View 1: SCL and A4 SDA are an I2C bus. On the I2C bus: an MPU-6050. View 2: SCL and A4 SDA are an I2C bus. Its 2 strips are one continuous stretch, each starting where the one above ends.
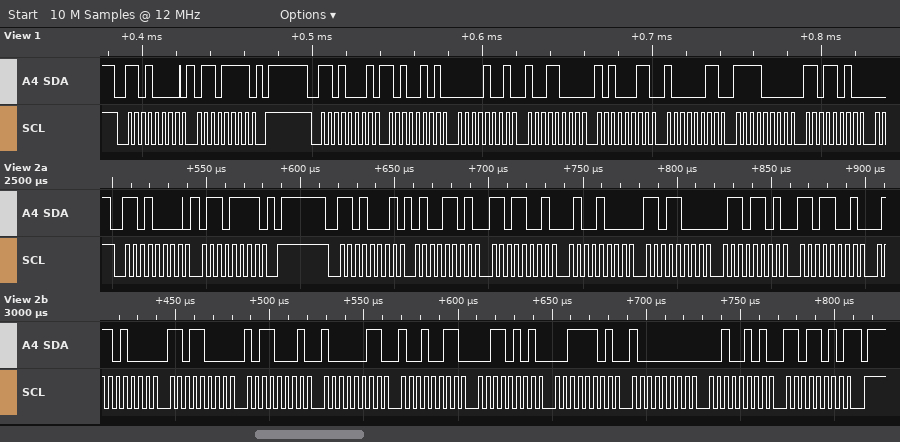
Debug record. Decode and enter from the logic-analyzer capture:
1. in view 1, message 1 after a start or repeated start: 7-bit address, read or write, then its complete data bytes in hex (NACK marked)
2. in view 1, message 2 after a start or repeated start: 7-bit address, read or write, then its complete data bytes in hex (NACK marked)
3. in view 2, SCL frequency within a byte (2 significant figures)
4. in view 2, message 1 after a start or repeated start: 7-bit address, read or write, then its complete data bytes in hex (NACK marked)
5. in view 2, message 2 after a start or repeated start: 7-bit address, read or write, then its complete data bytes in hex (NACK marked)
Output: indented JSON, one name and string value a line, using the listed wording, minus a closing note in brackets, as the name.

{
  "in view 1, message 1 after a start or repeated start: 7-bit address, read or write, then its complete data bytes in hex": "0x68 write: 6F",
  "in view 1, message 2 after a start or repeated start: 7-bit address, read or write, then its complete data bytes in hex": "0x68 read: A5 09 98 A3 83 F0 DA",
  "in view 2, SCL frequency within a byte": "250 kHz",
  "in view 2, message 1 after a start or repeated start: 7-bit address, read or write, then its complete data bytes in hex": "0x68 write: 6F",
  "in view 2, message 2 after a start or repeated start: 7-bit address, read or write, then its complete data bytes in hex": "0x68 read: 4D D9 48 D8 6D D9 68 D8 B1 83 93 35 3D 80 25 DA NACK"
}
